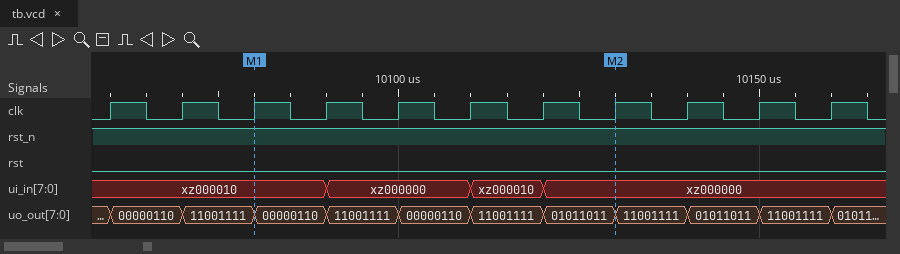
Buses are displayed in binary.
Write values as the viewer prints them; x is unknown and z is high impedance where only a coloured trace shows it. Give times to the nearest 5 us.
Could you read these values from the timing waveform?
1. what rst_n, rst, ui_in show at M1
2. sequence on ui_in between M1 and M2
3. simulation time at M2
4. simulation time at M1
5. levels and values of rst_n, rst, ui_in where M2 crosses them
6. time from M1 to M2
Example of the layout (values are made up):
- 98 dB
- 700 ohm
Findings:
- rst_n=1, rst=0, ui_in=xz000010
- xz000010, xz000000, xz000010, xz000000
- 10130 us
- 10080 us
- rst_n=1, rst=0, ui_in=xz000000
- 50 us
